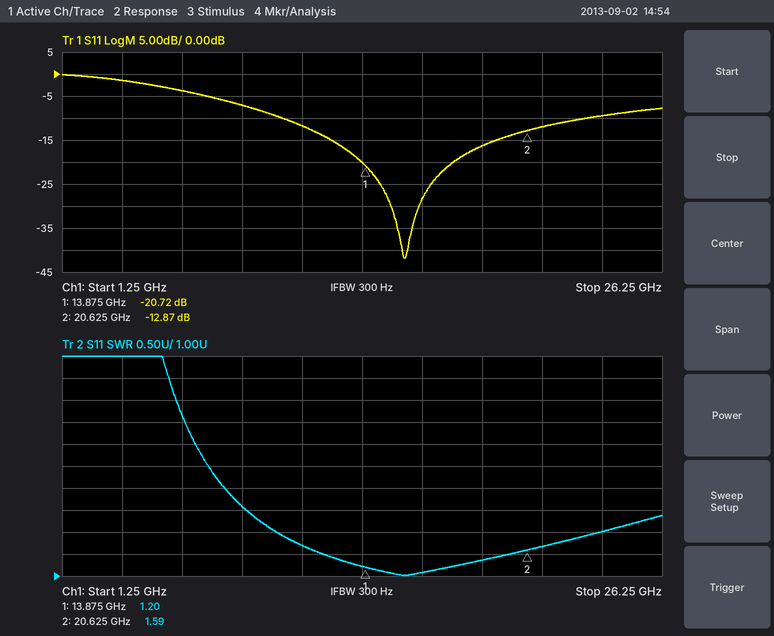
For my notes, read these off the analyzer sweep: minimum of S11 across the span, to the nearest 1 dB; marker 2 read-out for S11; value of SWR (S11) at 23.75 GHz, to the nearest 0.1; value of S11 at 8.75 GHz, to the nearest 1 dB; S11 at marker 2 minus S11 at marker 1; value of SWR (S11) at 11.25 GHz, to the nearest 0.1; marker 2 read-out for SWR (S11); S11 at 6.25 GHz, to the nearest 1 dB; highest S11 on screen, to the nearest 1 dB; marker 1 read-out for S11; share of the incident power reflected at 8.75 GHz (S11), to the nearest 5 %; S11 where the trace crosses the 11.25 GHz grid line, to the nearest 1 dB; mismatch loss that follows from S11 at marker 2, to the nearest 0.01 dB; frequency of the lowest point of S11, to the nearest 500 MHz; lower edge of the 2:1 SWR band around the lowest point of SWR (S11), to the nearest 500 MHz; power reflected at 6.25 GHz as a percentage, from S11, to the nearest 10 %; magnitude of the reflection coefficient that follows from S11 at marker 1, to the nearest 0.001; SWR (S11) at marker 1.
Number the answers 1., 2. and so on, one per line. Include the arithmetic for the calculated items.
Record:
1. -42 dB
2. -12.87 dB
3. 2.0
4. -7 dB
5. -12.87 − (-20.72) = 7.85 dB
6. 1.7
7. 1.59
8. -4 dB
9. 0 dB
10. -20.72 dB
11. 10^(-7/10) ≈ 20 %
12. -12 dB
13. −10 log10(1 − 10^(-12.87/10)) ≈ 0.23 dB
14. 15.5 GHz
15. 10.0 GHz
16. 10^(-4/10) ≈ 40 %
17. 10^(-20.72/20) ≈ 0.092
18. 1.20
